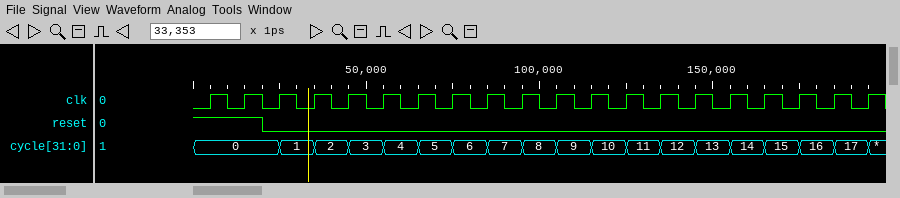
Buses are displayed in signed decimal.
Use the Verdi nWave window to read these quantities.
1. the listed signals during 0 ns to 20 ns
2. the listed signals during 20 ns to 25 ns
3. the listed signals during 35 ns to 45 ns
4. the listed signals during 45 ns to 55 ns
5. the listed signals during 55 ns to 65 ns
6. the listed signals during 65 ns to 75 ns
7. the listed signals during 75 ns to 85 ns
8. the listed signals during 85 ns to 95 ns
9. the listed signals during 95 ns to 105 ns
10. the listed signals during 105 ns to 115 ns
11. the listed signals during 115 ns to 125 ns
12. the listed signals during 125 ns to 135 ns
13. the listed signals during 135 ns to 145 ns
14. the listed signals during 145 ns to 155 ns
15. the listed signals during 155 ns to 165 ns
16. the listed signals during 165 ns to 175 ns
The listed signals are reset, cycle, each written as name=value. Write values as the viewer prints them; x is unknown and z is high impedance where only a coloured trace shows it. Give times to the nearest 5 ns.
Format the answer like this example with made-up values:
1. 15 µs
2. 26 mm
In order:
1. reset=1, cycle=0
2. reset=0, cycle=0
3. reset=0, cycle=2
4. reset=0, cycle=3
5. reset=0, cycle=4
6. reset=0, cycle=5
7. reset=0, cycle=6
8. reset=0, cycle=7
9. reset=0, cycle=8
10. reset=0, cycle=9
11. reset=0, cycle=10
12. reset=0, cycle=11
13. reset=0, cycle=12
14. reset=0, cycle=13
15. reset=0, cycle=14
16. reset=0, cycle=15
